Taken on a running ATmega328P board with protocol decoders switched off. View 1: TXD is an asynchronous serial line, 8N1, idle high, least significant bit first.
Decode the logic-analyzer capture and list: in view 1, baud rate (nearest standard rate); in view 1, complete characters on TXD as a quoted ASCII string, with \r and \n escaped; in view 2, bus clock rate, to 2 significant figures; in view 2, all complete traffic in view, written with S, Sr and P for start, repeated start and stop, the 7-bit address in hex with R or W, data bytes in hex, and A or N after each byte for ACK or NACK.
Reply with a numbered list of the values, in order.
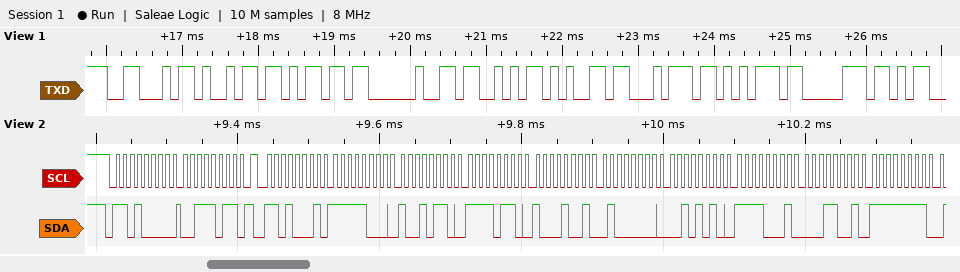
1. 9600 baud
2. "Fim Setup"
3. 100 kHz
4. S 68W A 3B A Sr 68R A F8 A 96 A F6 A 89 A 40 A 2A A F1 A 19 A FF A
